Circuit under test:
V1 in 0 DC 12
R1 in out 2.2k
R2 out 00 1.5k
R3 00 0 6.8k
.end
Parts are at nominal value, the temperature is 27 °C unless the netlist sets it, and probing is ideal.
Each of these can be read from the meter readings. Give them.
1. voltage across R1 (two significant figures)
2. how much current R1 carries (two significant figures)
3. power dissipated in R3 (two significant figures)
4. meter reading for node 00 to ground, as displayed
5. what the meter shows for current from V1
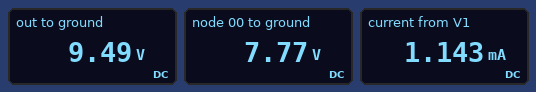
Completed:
2.5 V
1.1 mA
8.9 mW
7.77 V
1.143 mA
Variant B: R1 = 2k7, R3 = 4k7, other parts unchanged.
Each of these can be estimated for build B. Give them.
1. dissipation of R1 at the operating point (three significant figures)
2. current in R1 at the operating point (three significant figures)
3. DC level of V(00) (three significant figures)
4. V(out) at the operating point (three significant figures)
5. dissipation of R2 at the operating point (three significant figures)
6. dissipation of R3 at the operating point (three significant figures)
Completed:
4.91 mW
1.35 mA
6.34 V
8.36 V
2.73 mW
8.54 mW
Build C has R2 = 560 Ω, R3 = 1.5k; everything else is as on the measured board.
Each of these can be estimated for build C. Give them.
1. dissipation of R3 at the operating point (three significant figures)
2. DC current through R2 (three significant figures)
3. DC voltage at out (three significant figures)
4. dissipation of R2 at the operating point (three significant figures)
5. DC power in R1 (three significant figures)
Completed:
11.9 mW
2.82 mA
5.80 V
4.44 mW
17.5 mW
